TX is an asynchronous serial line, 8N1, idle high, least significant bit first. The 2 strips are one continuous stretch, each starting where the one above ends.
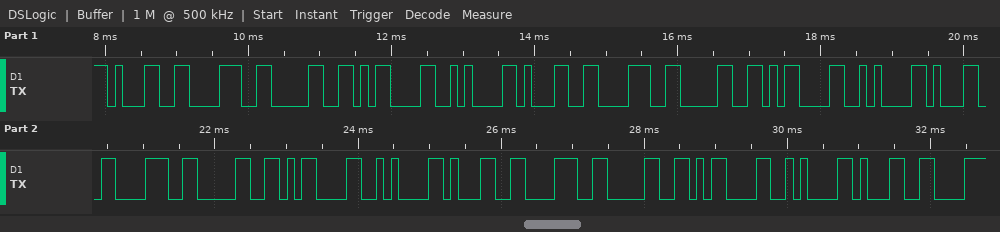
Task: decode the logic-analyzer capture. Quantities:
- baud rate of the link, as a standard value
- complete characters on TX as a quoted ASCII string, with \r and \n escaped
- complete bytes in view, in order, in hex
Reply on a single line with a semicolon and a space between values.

9600 baud; "180\r\n180\r\n180\r\n180\r\n1"; 31 38 30 0D 0A 31 38 30 0D 0A 31 38 30 0D 0A 31 38 30 0D 0A 31
